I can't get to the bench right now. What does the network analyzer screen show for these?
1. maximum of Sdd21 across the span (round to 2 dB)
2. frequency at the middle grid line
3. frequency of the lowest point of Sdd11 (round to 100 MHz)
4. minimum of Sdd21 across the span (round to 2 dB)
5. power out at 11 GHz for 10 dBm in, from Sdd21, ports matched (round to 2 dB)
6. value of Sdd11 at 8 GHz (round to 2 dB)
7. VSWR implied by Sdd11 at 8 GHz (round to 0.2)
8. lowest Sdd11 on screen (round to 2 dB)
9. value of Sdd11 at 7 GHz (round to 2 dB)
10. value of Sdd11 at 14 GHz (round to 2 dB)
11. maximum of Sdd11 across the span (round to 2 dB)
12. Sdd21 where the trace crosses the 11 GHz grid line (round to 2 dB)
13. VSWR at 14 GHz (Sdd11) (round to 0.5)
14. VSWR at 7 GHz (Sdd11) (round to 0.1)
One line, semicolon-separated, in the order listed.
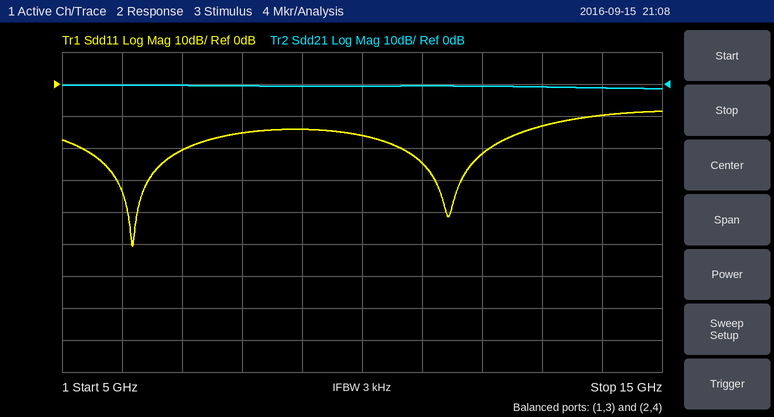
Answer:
0 dB; 10 GHz; 6.2 GHz; -2 dB; 10 dBm; -16 dB; 1.4; -50 dB; -20 dB; -10 dB; -8 dB; 0 dB; 2.0; 1.2
